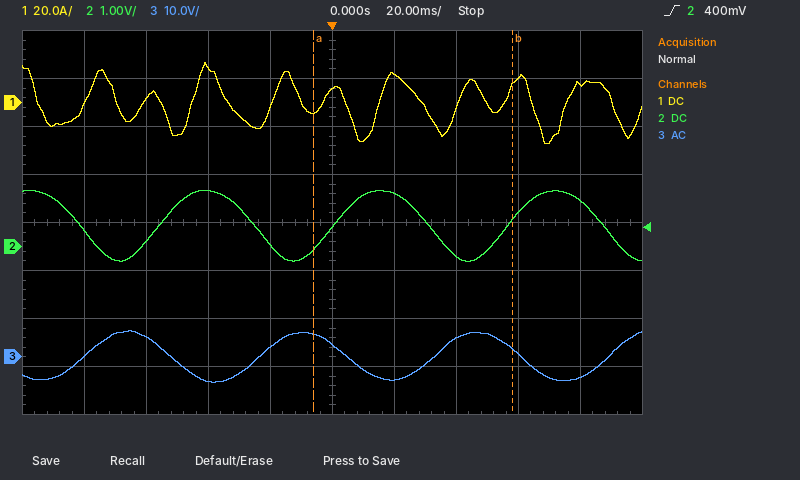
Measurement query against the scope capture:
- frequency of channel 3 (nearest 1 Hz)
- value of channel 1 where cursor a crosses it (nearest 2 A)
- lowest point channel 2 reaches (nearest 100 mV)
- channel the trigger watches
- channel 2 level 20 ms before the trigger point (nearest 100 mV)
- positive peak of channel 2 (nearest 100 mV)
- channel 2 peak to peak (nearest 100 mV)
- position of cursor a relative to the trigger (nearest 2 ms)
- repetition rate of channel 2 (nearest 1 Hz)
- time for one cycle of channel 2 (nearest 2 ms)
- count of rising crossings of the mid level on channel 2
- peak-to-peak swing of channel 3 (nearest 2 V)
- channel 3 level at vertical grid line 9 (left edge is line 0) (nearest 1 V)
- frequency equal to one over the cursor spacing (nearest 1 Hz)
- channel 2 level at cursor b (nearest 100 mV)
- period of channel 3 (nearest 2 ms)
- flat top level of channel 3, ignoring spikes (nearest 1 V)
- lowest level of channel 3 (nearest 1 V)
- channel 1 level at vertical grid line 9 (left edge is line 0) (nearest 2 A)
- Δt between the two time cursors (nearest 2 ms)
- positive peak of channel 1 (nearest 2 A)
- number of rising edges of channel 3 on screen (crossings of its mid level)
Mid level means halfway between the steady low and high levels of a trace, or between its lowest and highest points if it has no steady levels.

18 Hz
-4 A
-300 mV
channel 2
0.0 V
1.2 V
1.5 V
-6 ms
18 Hz
56 ms
3
10 V
-4 V
16 Hz
600 mV
56 ms
5 V
-5 V
8 A
64 ms
16 A
4
